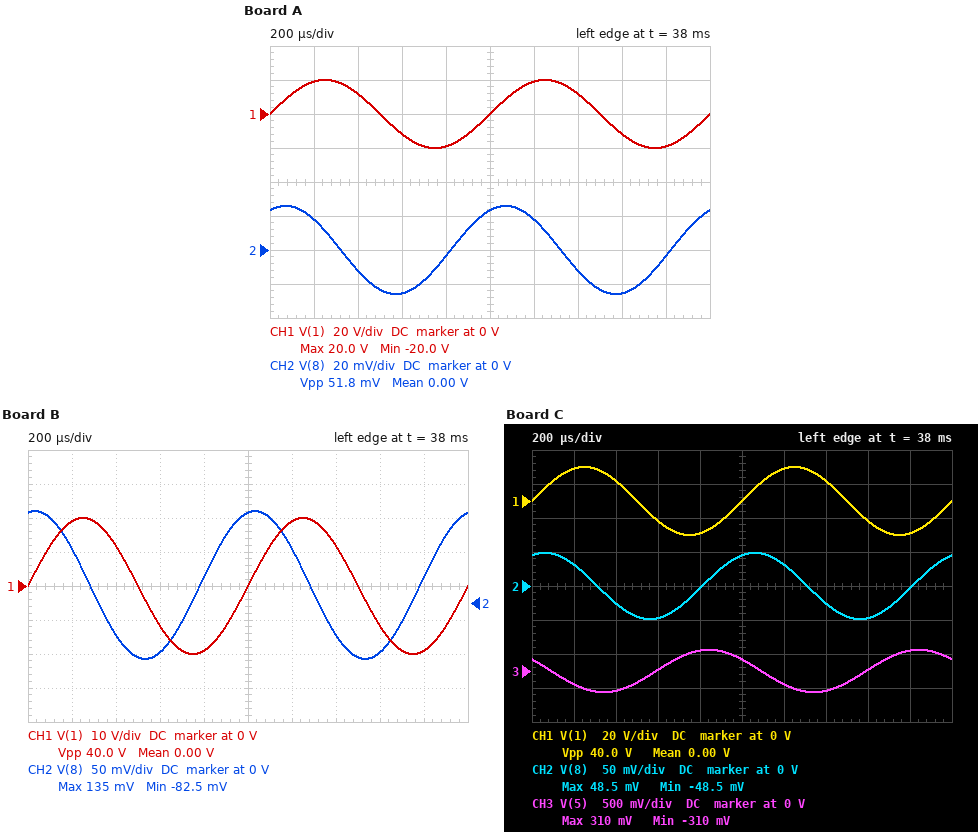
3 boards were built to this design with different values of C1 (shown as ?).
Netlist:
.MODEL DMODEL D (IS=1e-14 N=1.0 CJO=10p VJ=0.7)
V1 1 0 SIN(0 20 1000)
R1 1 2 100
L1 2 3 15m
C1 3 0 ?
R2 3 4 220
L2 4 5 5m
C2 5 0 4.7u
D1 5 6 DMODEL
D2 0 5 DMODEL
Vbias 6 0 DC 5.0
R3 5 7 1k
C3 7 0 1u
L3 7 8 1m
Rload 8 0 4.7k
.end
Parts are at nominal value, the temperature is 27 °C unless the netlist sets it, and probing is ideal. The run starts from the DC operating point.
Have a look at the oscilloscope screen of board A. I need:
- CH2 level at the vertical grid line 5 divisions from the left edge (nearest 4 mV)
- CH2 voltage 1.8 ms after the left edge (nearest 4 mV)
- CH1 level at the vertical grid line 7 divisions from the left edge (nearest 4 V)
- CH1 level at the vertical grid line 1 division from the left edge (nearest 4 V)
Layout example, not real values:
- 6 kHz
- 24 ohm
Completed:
- 24 mV
- -4 mV
- 12 V
- 20 V
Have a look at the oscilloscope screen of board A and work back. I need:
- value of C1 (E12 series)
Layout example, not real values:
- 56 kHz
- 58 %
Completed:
- 22 µF
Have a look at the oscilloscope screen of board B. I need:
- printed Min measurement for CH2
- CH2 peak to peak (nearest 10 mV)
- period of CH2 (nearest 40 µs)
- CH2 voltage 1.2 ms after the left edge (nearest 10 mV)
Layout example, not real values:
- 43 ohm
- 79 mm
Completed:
- -82.5 mV
- 220 mV
- 1.00 ms
- 80 mV
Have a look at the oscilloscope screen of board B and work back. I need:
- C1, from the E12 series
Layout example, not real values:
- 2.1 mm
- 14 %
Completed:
- 5.6 µF
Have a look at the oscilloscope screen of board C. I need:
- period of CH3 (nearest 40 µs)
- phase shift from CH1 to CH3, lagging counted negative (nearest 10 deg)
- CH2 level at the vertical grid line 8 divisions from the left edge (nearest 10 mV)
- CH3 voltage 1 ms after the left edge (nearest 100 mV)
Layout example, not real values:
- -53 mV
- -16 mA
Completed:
- 1.00 ms
- 150 deg
- -50 mV
- 200 mV
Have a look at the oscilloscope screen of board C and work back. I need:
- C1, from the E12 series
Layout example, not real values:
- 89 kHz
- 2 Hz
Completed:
- 12 µF
